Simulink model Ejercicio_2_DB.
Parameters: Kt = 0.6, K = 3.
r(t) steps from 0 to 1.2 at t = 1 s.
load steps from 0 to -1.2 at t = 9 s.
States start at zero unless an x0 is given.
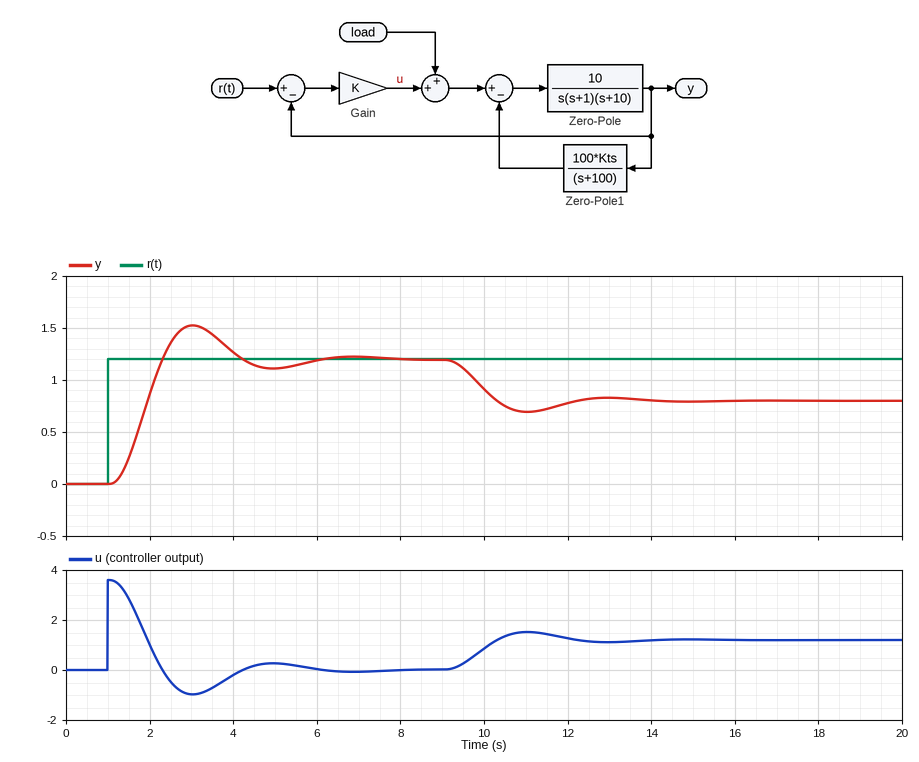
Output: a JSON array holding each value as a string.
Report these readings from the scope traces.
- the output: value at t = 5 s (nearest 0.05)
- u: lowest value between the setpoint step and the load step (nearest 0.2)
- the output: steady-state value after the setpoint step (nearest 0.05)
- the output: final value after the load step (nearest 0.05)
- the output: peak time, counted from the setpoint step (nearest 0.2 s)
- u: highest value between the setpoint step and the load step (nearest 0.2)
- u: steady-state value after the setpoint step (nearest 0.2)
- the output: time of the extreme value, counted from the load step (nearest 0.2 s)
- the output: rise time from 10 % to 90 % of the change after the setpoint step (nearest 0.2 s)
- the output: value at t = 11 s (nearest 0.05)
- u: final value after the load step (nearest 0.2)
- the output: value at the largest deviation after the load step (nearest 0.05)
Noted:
["1.10", "-1.0", "1.20", "0.80", "2.0 s", "3.6", "0.0", "2.0 s", "0.8 s", "0.70", "1.2", "0.70"]
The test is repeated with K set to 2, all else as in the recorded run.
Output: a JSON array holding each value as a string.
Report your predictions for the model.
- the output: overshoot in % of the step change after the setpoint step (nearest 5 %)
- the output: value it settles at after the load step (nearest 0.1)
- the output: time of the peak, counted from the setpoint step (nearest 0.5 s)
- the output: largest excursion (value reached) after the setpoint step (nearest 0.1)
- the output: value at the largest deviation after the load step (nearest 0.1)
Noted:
["15 %", "0.6", "2.5 s", "1.4", "0.5"]
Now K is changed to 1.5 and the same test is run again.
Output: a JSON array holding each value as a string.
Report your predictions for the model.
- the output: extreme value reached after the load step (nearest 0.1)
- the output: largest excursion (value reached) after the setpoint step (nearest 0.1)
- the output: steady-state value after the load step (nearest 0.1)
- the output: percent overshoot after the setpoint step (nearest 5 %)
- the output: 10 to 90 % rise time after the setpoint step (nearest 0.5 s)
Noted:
["0.3", "1.3", "0.4", "10 %", "1.5 s"]
